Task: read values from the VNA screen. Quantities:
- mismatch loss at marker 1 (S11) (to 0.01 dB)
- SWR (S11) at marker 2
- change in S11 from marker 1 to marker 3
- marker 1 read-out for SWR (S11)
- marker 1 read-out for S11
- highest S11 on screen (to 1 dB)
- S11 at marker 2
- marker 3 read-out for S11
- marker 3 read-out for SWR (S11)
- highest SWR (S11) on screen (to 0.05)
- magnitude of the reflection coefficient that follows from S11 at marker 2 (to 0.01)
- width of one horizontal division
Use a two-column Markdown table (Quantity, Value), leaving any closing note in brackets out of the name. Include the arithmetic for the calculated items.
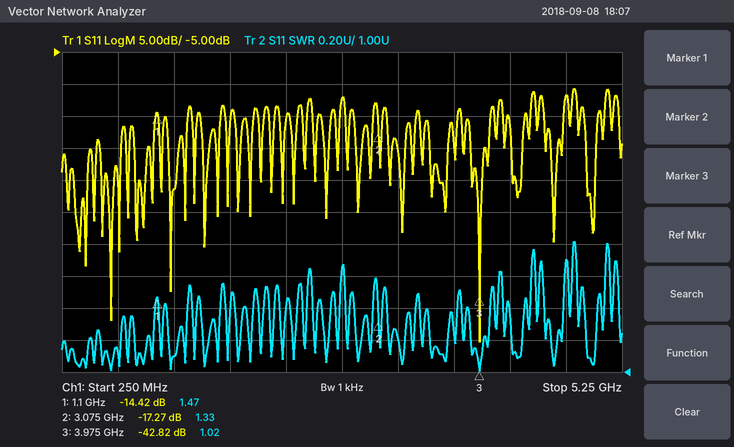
| Quantity | Value |
|---|---|
| mismatch loss at marker 1 (S11) | −10 log10(1 − 10^(-14.42/10)) ≈ 0.16 dB |
| SWR (S11) at marker 2 | 1.33 |
| change in S11 from marker 1 to marker 3 | -42.82 − (-14.42) = -28.40 dB |
| marker 1 read-out for SWR | 1.47 |
| marker 1 read-out for S11 | -14.42 dB |
| highest S11 on screen | -11 dB |
| S11 at marker 2 | -17.27 dB |
| marker 3 read-out for S11 | -42.82 dB |
| marker 3 read-out for SWR | 1.02 |
| highest SWR (S11) on screen | 1.80 |
| magnitude of the reflection coefficient that follows from S11 at marker 2 | 10^(-17.27/20) ≈ 0.14 |
| width of one horizontal division | 500 MHz |
